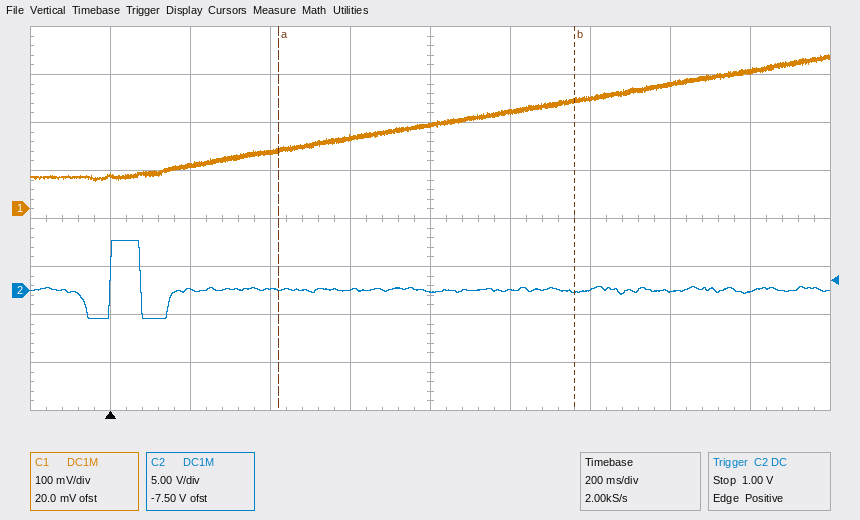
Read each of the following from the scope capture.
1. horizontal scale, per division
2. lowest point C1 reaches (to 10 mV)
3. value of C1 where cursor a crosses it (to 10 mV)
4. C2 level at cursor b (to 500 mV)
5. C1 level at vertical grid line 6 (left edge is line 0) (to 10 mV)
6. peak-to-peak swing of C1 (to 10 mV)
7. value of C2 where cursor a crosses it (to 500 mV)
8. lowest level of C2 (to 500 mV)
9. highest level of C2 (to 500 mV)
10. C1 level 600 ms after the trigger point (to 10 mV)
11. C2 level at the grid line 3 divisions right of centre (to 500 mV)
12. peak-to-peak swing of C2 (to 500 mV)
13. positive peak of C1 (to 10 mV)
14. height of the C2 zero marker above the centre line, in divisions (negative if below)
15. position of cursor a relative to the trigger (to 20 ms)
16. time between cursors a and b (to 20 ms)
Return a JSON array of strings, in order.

["200 ms", "60 mV", "120 mV", "0.0 V", "200 mV", "260 mV", "0.0 V", "-3.0 V", "5.0 V", "150 mV", "0.0 V", "8.0 V", "320 mV", "-1.5 div", "+420 ms", "740 ms"]
